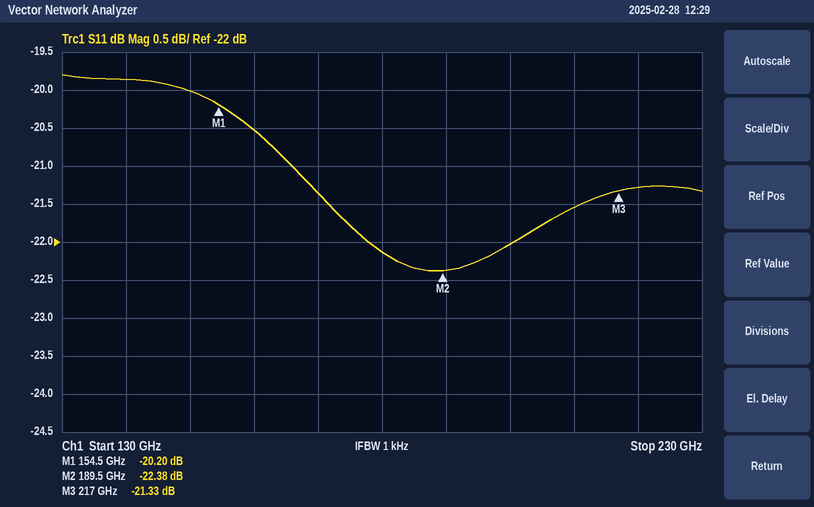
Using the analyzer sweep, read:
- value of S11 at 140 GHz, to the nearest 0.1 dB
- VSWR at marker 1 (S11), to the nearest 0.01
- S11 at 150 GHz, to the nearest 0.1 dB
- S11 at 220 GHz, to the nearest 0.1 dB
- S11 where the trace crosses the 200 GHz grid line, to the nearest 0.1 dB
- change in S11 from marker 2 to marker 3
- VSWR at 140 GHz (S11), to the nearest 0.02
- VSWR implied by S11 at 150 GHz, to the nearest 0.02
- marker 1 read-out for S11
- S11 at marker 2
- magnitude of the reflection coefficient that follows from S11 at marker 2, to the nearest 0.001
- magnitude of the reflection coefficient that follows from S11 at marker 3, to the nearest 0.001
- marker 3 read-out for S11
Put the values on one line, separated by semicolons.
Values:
-19.9 dB; 1.22; -20.0 dB; -21.3 dB; -22.0 dB; 1.05 dB; 1.22; 1.22; -20.20 dB; -22.38 dB; 0.076; 0.086; -21.33 dB
